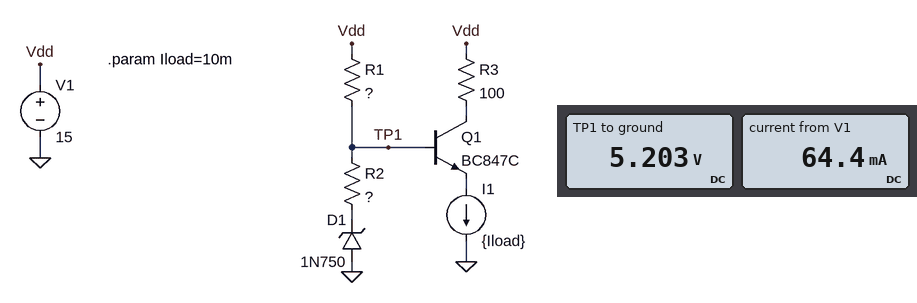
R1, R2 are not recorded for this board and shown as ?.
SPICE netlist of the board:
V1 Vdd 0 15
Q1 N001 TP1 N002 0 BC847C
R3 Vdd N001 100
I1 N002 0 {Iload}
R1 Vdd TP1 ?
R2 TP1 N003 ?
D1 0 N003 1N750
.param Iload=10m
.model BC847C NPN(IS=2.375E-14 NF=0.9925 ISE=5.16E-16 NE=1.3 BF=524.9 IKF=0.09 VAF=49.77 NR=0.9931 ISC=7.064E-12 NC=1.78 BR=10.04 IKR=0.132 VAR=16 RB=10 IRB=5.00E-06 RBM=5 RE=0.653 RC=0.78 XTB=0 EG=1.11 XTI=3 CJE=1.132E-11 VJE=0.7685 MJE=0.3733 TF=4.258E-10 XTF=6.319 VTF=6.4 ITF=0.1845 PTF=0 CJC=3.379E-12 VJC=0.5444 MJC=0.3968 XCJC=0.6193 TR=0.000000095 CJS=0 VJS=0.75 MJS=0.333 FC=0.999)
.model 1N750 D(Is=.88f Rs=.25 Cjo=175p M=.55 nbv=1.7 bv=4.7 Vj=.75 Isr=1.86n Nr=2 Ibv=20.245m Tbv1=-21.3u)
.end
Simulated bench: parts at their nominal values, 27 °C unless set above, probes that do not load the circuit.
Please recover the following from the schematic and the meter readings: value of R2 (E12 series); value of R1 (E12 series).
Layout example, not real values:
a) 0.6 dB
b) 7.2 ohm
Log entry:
a) 8.2 Ω
b) 180 Ω
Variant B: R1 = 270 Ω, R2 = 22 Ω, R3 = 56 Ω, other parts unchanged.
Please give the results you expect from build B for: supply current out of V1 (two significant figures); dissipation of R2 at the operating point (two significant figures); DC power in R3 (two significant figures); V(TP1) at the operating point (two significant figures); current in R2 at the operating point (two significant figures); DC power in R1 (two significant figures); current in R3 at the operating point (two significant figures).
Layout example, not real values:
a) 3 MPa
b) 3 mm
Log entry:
a) 45 mA
b) 27 mW
c) 5.6 mW
d) 5.5 V
e) 35 mA
f) 330 mW
g) 10 mA
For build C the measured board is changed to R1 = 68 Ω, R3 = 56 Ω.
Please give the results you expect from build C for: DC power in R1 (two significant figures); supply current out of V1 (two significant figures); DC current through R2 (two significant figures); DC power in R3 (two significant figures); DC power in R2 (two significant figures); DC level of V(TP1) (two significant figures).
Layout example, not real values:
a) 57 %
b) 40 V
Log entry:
a) 1.2 W
b) 140 mA
c) 130 mA
d) 5.6 mW
e) 150 mW
f) 5.9 V
